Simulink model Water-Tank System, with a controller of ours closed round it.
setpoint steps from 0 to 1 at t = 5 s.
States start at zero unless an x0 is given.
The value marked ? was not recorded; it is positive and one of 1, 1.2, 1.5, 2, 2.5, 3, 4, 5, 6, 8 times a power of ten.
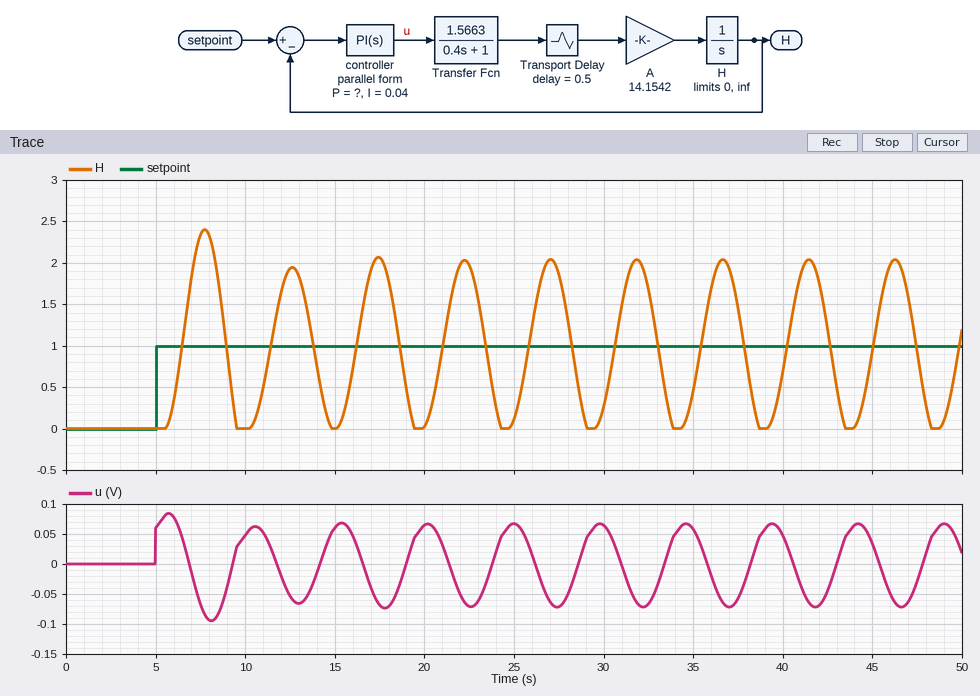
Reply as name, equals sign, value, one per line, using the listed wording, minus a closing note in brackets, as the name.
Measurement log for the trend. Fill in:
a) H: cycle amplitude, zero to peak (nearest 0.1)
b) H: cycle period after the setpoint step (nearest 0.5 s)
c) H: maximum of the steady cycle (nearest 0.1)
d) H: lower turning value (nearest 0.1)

H: cycle amplitude, zero to peak = 1.0
H: cycle period after the setpoint step = 5.0 s
H: maximum of the steady cycle = 2.0
H: lower turning value = 0.0
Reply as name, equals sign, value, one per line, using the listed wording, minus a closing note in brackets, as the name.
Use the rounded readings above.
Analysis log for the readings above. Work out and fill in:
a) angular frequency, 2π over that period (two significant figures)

angular frequency, 2π over that period = 1.3 rad/s
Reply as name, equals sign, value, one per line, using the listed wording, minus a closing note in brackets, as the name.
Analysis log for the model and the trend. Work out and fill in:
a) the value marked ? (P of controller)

the value marked ? = 0.06
